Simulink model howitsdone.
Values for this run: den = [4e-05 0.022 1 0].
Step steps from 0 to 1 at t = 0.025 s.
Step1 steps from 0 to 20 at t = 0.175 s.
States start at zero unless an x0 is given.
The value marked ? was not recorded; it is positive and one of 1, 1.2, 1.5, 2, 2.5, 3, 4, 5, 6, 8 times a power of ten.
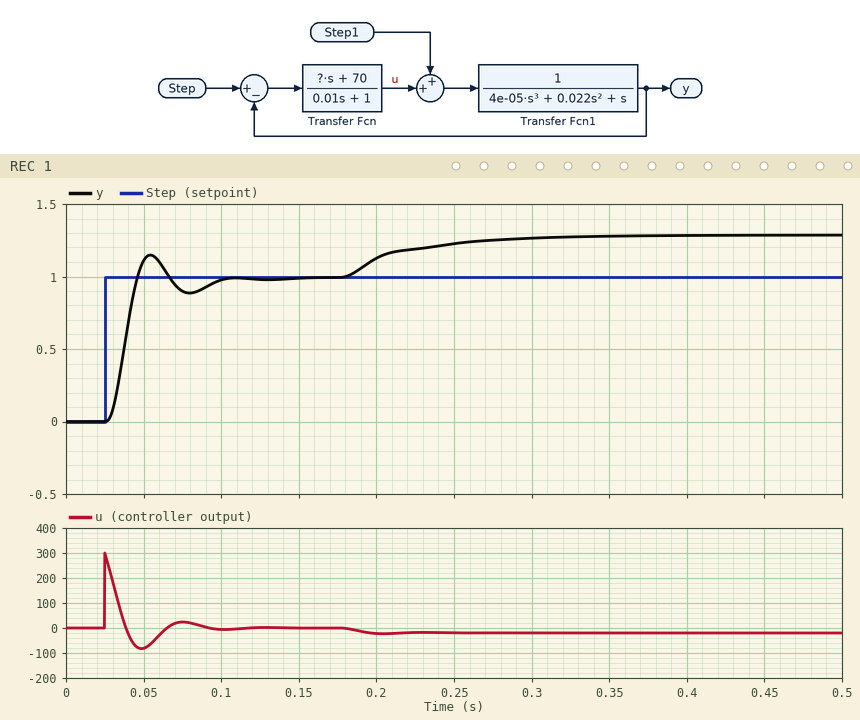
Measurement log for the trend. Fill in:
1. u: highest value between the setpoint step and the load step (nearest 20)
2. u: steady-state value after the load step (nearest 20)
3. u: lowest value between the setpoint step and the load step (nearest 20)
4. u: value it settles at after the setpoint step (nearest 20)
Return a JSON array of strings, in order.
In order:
["300", "-20", "-80", "0"]
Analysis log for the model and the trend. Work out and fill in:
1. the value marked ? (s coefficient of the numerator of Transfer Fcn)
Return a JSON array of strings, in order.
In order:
["3"]
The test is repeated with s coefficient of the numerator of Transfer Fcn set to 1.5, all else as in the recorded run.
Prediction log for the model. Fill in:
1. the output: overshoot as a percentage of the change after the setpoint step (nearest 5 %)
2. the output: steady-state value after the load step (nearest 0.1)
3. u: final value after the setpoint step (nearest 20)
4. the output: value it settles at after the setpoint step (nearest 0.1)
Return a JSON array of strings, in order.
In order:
["15 %", "1.3", "0", "1.0"]
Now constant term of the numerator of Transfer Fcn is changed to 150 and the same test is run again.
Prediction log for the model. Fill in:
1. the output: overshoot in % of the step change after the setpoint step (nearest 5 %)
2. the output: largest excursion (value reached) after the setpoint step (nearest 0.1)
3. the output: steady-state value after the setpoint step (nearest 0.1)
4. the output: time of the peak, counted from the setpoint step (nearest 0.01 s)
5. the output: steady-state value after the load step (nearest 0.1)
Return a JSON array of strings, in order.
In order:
["40 %", "1.4", "1.0", "0.03 s", "1.1"]
